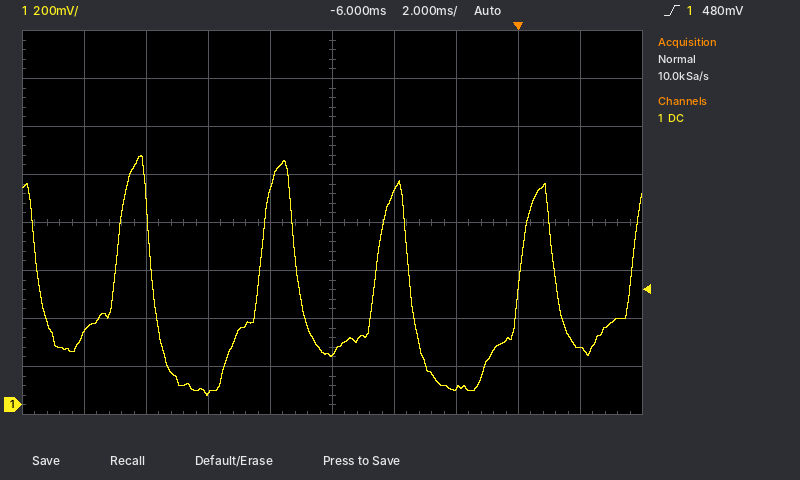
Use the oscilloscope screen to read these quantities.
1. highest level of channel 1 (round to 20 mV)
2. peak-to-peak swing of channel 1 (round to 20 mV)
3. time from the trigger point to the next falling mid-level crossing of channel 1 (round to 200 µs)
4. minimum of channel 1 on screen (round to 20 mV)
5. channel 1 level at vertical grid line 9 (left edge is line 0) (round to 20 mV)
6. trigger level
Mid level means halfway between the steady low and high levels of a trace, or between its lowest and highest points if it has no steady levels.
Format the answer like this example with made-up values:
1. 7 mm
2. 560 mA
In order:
1. 1.04 V
2. 1.00 V
3. 1.2 ms
4. 40 mV
5. 240 mV
6. 480 mV
